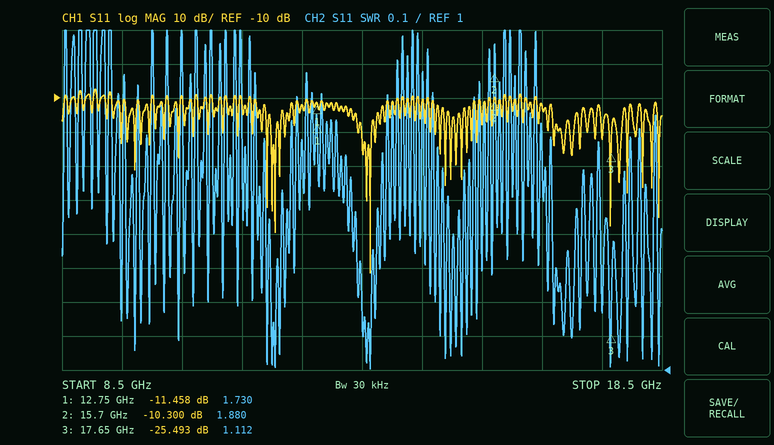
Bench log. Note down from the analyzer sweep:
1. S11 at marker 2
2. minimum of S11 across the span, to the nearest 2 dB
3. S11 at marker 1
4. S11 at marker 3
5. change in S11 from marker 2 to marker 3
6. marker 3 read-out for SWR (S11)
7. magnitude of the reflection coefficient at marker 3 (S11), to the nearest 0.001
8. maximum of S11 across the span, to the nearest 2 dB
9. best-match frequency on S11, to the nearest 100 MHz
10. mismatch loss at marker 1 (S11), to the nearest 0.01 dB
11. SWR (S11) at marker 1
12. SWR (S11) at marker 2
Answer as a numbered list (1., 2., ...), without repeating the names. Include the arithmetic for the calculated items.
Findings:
1. -10.300 dB
2. -62 dB
3. -11.458 dB
4. -25.493 dB
5. -25.493 − (-10.3) = -15.193 dB
6. 1.112
7. 10^(-25.493/20) ≈ 0.053
8. -8 dB
9. 13.6 GHz
10. −10 log10(1 − 10^(-11.458/10)) ≈ 0.32 dB
11. 1.730
12. 1.880
